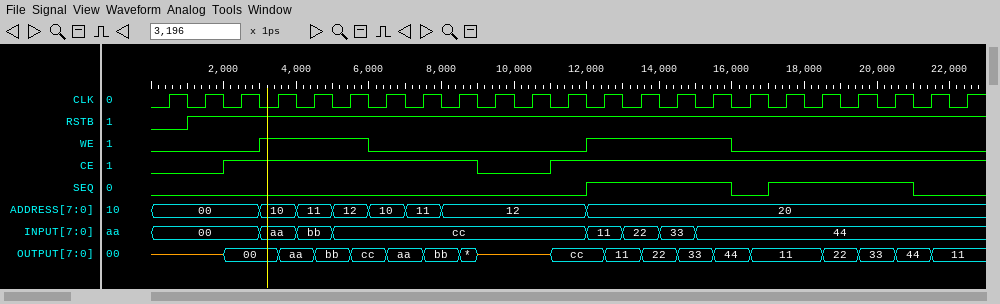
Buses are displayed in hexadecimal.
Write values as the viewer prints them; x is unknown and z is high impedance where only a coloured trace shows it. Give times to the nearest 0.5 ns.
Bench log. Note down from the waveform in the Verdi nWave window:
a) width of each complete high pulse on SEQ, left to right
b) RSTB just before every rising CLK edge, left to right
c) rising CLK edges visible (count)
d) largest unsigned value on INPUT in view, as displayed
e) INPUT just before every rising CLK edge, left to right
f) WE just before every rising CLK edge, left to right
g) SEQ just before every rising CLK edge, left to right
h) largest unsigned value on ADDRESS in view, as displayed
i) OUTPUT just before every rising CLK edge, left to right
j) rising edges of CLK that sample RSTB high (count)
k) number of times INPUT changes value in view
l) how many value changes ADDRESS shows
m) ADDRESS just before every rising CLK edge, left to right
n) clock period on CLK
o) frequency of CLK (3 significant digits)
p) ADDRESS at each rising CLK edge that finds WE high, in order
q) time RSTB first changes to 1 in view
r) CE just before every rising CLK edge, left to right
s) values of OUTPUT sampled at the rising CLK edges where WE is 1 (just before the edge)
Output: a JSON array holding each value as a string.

["4 ns, 4 ns", "0 1 1 1 1 1 1 1 1 1 1 1 1 1 1 1 1 1 1 1 1 1 1", "23", "cc", "00, 00, 00, aa, bb, cc, cc, cc, cc, cc, cc, cc, 11, 22, 33, 44, 44, 44, 44, 44, 44, 44, 44", "0 0 0 1 1 1 0 0 0 0 0 0 1 1 1 1 0 0 0 0 0 0 0", "0 0 0 0 0 0 0 0 0 0 0 0 1 1 1 1 0 1 1 1 1 0 0", "20", "z, z, 00, 00, aa, bb, cc, aa, bb, z, z, cc, cc, 11, 22, 33, 44, 11, 11, 22, 33, 44, 11", "22", "7", "7", "00, 00, 00, 10, 11, 12, 10, 11, 12, 12, 12, 12, 20, 20, 20, 20, 20, 20, 20, 20, 20, 20, 20", "1 ns", "1.00 GHz", "10, 11, 12, 20, 20, 20, 20", "1 ns", "0 0 1 1 1 1 1 1 1 0 0 1 1 1 1 1 1 1 1 1 1 1 1", "00, aa, bb, cc, 11, 22, 33"]
